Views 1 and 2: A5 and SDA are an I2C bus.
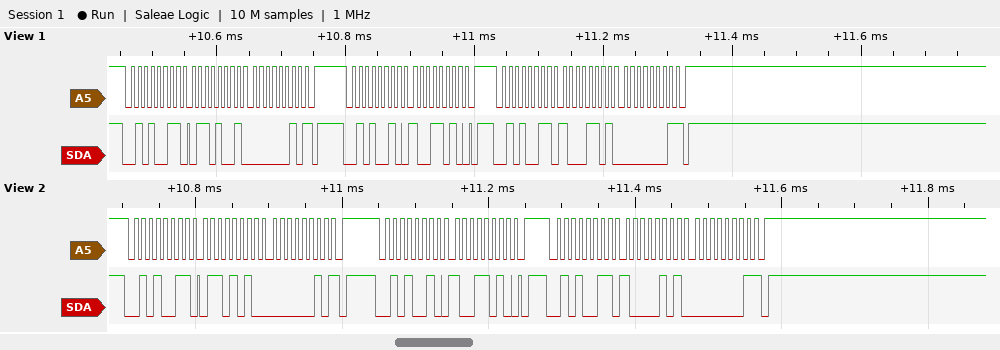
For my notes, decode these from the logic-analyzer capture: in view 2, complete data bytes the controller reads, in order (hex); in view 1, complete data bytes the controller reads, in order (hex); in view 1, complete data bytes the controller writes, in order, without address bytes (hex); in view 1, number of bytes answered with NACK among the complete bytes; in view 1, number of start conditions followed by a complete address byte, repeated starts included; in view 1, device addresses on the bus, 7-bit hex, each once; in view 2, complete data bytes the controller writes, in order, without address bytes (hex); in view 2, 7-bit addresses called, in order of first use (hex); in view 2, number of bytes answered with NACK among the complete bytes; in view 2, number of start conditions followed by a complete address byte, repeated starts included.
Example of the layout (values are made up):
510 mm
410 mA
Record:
6A 02 85 01
69 02 8D 01
9A
2
3
0x29
9A
0x29
2
3
